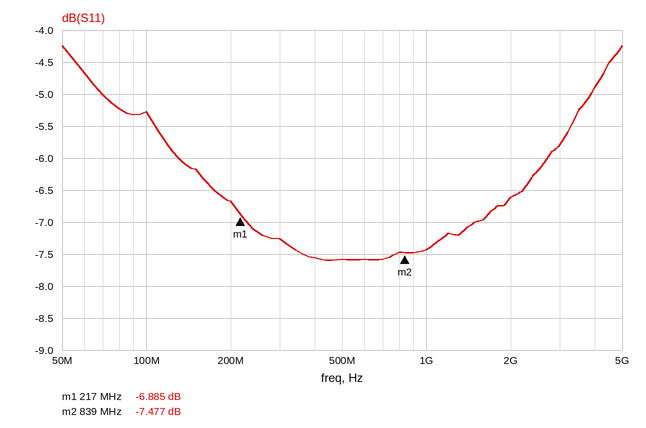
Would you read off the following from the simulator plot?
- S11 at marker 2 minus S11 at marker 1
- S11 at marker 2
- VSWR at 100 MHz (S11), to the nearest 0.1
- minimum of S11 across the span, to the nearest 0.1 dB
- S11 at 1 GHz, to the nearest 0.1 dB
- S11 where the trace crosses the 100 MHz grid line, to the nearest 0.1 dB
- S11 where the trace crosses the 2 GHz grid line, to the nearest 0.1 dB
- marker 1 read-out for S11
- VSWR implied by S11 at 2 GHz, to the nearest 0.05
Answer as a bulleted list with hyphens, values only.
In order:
- -0.592 dB
- -7.477 dB
- 3.4
- -7.6 dB
- -7.4 dB
- -5.3 dB
- -6.6 dB
- -6.885 dB
- 2.75
